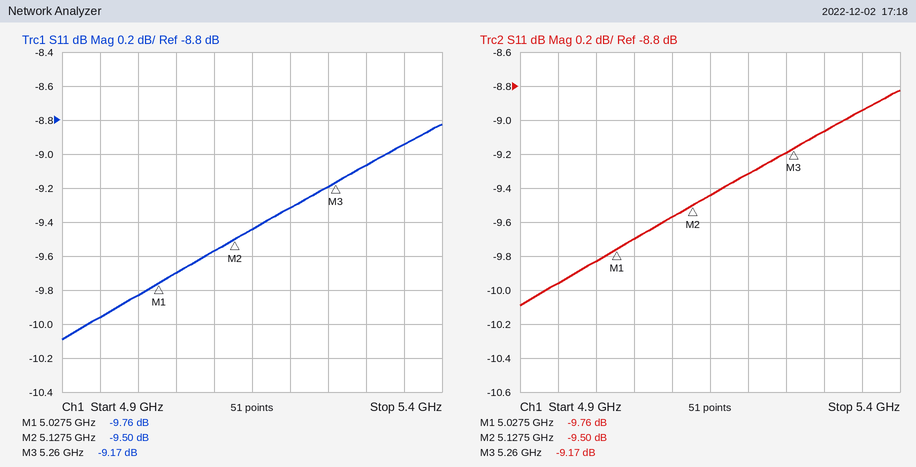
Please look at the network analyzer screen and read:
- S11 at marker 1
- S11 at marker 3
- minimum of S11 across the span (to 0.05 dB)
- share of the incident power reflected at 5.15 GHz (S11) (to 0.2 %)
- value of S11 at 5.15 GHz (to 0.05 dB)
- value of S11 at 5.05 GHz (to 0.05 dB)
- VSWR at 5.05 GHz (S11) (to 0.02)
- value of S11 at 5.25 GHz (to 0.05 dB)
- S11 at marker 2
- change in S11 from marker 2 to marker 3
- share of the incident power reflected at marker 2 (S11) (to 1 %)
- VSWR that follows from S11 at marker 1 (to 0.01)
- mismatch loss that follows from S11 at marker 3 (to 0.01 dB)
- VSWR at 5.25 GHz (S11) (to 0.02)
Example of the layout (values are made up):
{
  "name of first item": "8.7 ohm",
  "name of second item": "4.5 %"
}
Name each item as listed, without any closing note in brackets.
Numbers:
{
  "S11 at marker 1": "-9.76 dB",
  "S11 at marker 3": "-9.17 dB",
  "minimum of S11 across the span": "-10.10 dB",
  "share of the incident power reflected at 5.15 GHz (S11)": "11.4 %",
  "value of S11 at 5.15 GHz": "-9.45 dB",
  "value of S11 at 5.05 GHz": "-9.70 dB",
  "VSWR at 5.05 GHz (S11)": "1.98",
  "value of S11 at 5.25 GHz": "-9.20 dB",
  "S11 at marker 2": "-9.50 dB",
  "change in S11 from marker 2 to marker 3": "0.33 dB",
  "share of the incident power reflected at marker 2 (S11)": "11 %",
  "VSWR that follows from S11 at marker 1": "1.96",
  "mismatch loss that follows from S11 at marker 3": "0.56 dB",
  "VSWR at 5.25 GHz (S11)": "2.06"
}
